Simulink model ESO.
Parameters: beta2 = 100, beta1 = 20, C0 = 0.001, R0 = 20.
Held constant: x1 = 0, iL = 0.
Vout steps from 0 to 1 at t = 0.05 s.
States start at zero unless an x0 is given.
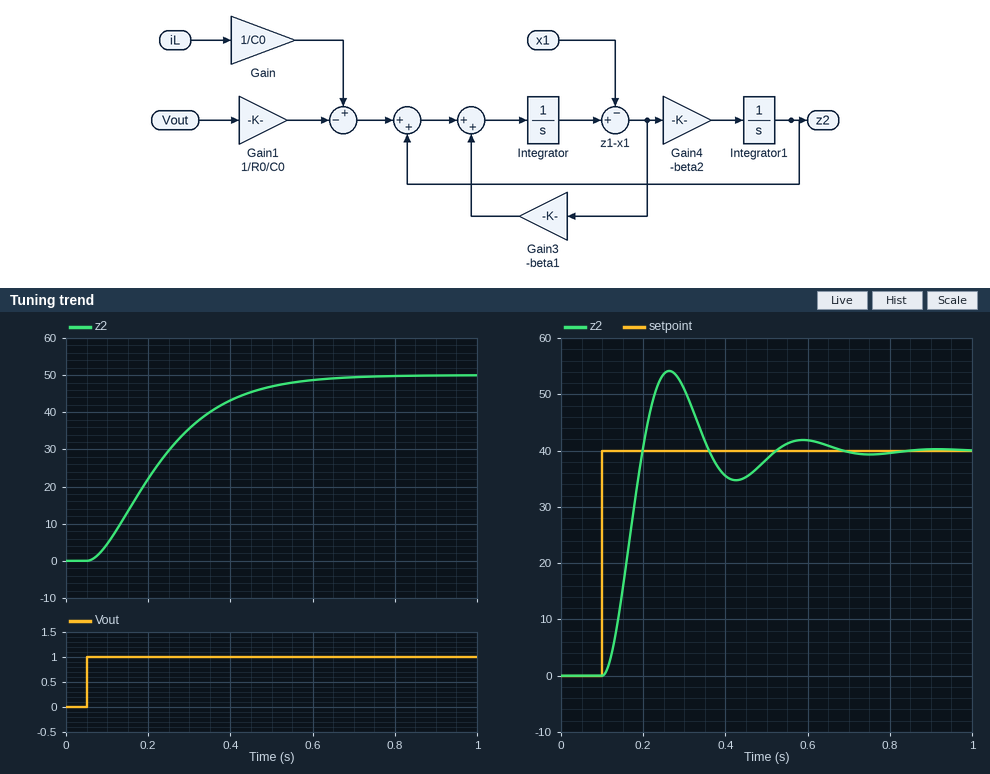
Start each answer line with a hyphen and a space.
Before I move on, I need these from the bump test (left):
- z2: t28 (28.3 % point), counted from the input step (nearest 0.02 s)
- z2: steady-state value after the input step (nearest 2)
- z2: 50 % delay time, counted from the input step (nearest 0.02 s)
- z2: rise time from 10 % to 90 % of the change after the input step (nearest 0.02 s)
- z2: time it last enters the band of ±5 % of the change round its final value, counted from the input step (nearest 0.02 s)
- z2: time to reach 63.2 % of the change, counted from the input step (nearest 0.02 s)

- 0.10 s
- 50
- 0.16 s
- 0.34 s
- 0.48 s
- 0.22 s
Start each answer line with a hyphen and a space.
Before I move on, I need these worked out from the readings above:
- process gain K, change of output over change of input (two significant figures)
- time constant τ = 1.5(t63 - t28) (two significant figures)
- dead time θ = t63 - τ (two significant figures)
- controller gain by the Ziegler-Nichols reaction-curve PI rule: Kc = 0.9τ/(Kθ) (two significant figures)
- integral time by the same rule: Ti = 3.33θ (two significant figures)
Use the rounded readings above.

- 50
- 0.18 s
- 0.040 s
- 0.081
- 0.13 s
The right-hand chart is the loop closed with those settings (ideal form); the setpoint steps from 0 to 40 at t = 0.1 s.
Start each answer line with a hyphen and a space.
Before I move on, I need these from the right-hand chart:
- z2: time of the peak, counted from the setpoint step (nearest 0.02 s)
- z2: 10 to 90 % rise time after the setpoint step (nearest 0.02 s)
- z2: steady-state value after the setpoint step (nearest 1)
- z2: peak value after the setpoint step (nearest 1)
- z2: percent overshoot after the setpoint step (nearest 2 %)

- 0.16 s
- 0.06 s
- 40
- 54
- 36 %
